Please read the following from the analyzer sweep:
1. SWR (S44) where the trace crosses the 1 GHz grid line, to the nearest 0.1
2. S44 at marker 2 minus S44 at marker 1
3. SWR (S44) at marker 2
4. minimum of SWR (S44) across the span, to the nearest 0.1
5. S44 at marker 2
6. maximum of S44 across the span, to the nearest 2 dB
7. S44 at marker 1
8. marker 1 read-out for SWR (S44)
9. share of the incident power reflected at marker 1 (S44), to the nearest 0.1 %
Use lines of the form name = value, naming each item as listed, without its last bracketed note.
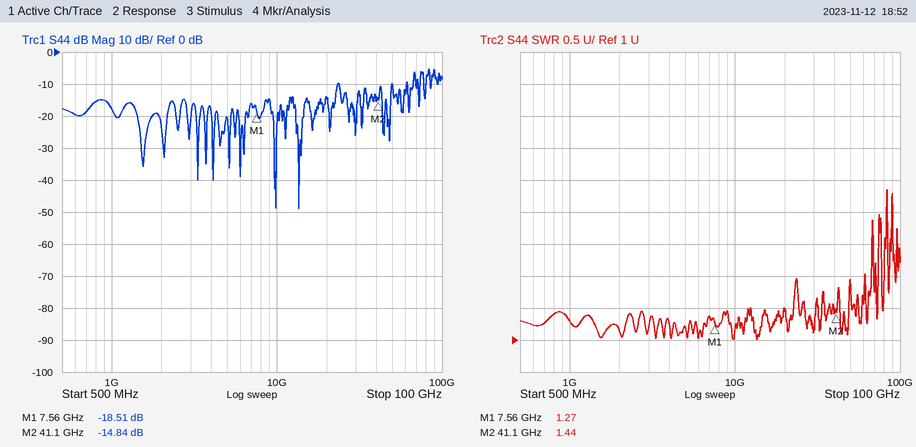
SWR (S44) where the trace crosses the 1 GHz grid line, to the nearest 0.1 = 1.3
S44 at marker 2 minus S44 at marker 1 = 3.67 dB
SWR (S44) at marker 2 = 1.44
minimum of SWR (S44) across the span, to the nearest 0.1 = 1.0
S44 at marker 2 = -14.84 dB
maximum of S44 across the span, to the nearest 2 dB = -6 dB
S44 at marker 1 = -18.51 dB
marker 1 read-out for SWR = 1.27
share of the incident power reflected at marker 1 (S44), to the nearest 0.1 % = 1.4 %
